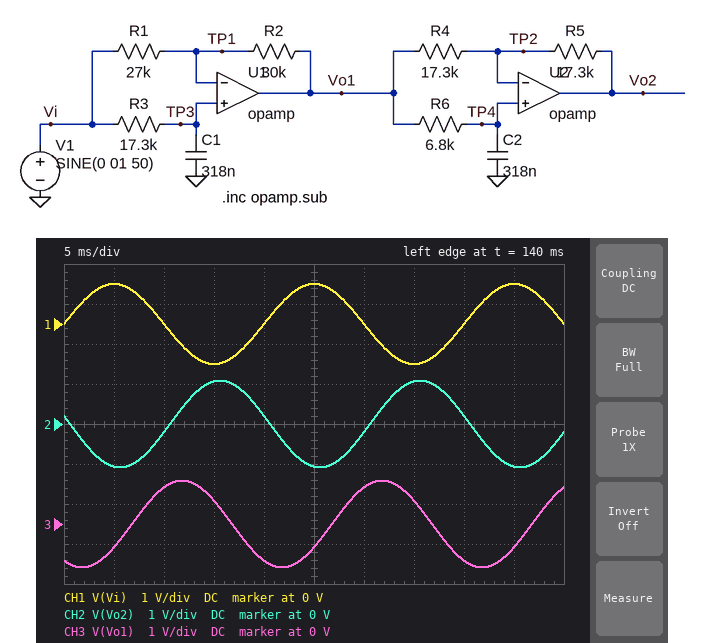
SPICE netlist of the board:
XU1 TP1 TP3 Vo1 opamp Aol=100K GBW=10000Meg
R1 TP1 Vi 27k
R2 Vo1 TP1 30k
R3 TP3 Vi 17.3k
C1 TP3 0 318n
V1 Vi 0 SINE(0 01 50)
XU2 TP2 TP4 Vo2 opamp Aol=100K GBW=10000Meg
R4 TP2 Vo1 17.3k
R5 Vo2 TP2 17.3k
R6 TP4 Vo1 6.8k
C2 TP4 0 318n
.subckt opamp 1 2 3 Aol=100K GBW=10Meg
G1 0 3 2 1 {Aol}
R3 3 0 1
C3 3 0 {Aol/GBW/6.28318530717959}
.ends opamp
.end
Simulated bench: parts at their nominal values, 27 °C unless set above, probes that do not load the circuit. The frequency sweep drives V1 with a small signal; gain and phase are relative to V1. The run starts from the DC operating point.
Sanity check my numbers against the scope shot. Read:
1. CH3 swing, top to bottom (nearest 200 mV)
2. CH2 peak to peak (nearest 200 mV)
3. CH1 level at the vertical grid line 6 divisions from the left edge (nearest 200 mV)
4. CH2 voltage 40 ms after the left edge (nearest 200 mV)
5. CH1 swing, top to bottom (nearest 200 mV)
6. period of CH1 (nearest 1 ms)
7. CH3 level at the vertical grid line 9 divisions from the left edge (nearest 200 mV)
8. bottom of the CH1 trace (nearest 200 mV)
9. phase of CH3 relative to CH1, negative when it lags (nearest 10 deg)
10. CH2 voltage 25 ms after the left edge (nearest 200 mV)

2.2 V
2.2 V
0 V
200 mV
2.0 V
20 ms
-600 mV
-1.0 V
-120 deg
-1.0 V
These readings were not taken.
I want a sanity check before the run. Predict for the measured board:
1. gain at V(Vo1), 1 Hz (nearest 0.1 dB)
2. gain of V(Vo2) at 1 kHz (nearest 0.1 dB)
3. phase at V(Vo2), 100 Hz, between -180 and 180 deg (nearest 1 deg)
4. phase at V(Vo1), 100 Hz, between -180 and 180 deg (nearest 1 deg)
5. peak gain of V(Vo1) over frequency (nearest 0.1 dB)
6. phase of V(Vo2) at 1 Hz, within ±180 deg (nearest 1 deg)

0 dB
0.9 dB
103 deg
-149 deg
0.9 dB
-6 deg
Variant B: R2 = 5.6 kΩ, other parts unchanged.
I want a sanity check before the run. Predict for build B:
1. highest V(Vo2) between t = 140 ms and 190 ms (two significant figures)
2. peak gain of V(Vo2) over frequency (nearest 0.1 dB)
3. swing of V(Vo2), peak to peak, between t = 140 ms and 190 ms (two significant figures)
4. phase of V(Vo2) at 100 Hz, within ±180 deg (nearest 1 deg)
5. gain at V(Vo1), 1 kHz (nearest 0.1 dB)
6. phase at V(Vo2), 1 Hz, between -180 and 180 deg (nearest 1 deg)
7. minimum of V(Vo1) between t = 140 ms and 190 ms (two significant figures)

530 mV
0 dB
1.1 V
143 deg
-13.6 dB
-4 deg
-530 mV
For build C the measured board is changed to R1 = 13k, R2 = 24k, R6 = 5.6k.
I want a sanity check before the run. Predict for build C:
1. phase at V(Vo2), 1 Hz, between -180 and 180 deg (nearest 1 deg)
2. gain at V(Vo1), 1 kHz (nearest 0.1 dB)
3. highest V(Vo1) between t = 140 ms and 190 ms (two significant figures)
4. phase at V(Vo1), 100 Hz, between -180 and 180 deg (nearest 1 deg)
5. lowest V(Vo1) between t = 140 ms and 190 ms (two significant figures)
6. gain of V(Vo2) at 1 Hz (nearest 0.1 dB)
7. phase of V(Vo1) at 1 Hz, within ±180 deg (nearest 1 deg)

-7 deg
5.3 dB
1.7 V
-155 deg
-1.7 V
0 dB
-6 deg
